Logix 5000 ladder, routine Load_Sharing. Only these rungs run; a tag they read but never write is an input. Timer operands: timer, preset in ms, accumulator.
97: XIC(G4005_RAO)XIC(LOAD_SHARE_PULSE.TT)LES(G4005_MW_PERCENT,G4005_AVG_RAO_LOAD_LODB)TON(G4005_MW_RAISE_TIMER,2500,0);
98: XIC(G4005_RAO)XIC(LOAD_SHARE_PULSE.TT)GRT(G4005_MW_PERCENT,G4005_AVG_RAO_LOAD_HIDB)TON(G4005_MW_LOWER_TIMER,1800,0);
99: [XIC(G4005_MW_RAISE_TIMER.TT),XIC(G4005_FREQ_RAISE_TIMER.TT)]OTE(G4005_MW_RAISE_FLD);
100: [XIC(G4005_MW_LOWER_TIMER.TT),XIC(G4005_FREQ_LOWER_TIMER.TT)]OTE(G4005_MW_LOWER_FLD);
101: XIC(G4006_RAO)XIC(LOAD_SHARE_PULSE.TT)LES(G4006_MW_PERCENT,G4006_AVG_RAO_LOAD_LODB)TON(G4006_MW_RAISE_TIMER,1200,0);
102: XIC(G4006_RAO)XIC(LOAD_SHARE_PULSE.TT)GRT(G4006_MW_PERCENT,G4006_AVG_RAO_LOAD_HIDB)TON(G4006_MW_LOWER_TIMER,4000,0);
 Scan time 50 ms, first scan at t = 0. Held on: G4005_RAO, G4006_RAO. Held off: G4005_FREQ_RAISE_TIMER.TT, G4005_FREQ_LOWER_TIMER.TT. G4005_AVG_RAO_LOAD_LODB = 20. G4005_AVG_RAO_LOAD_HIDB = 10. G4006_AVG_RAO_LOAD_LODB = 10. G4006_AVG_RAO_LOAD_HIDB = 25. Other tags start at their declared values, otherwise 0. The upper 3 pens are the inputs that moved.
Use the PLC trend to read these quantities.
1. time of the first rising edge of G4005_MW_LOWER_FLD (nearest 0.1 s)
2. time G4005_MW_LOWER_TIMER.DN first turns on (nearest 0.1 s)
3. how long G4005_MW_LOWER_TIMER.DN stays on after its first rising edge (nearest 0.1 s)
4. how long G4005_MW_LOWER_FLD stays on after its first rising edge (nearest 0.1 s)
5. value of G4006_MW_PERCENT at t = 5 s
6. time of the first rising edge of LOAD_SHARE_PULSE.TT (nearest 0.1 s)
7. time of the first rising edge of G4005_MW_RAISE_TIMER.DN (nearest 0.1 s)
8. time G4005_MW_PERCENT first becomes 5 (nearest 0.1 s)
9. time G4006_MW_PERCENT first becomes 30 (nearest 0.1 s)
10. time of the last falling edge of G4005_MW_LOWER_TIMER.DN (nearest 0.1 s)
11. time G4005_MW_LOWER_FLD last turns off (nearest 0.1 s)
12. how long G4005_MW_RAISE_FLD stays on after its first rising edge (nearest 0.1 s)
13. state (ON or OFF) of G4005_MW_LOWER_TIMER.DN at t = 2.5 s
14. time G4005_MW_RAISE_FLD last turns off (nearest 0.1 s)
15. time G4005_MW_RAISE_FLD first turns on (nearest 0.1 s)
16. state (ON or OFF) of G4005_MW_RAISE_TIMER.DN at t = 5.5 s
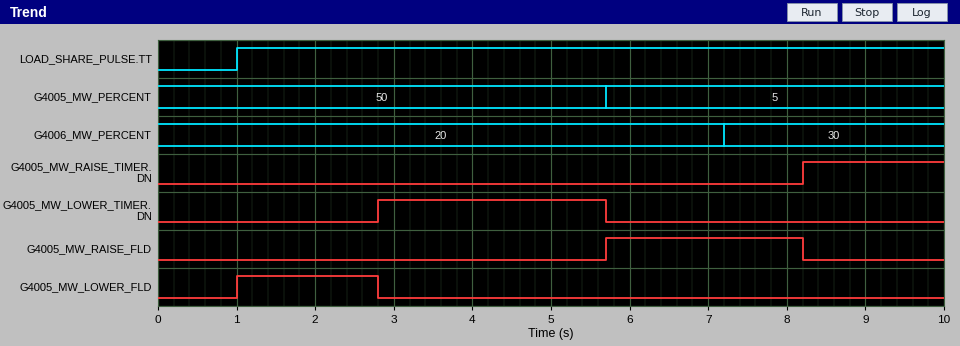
1.0 s
2.8 s
2.9 s
1.8 s
20
1.0 s
8.2 s
5.7 s
7.2 s
5.7 s
2.8 s
2.5 s
OFF
8.2 s
5.7 s
OFF
